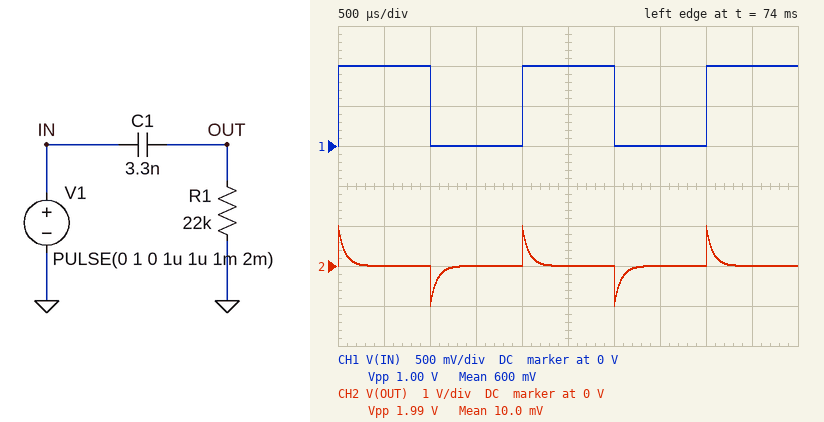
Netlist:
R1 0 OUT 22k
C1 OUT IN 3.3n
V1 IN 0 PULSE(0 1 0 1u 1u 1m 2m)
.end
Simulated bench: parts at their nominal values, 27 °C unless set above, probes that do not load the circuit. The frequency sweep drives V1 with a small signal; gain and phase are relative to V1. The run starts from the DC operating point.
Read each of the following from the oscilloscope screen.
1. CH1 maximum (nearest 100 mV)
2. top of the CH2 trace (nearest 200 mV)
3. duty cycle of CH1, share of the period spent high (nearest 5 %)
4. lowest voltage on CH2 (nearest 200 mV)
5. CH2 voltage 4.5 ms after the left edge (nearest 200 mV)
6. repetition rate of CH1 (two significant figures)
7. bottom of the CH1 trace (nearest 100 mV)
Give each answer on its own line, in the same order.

1.0 V
1.0 V
50 %
-1.0 V
0 V
500 Hz
0 V
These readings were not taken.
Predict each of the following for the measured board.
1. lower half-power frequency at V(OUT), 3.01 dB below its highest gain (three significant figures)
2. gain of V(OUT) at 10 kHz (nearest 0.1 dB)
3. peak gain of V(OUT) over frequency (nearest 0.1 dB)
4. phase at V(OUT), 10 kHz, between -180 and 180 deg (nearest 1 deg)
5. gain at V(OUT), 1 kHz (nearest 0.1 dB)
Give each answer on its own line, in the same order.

2.19 kHz
-0.2 dB
0 dB
12 deg
-7.6 dB
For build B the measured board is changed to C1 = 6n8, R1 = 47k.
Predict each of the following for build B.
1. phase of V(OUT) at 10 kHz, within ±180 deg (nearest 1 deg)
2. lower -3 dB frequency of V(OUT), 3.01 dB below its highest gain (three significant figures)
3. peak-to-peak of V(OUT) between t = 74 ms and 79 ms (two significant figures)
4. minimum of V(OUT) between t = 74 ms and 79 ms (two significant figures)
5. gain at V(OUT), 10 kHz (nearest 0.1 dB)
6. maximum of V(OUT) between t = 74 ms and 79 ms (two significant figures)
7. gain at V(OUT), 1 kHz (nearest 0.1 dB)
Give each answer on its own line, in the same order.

3 deg
498 Hz
1.9 V
-960 mV
0 dB
960 mV
-1.0 dB
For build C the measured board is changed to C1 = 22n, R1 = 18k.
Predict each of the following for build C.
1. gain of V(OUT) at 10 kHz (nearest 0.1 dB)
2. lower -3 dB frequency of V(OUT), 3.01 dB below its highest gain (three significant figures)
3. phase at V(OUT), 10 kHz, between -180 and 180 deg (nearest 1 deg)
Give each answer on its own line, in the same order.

0 dB
402 Hz
2 deg
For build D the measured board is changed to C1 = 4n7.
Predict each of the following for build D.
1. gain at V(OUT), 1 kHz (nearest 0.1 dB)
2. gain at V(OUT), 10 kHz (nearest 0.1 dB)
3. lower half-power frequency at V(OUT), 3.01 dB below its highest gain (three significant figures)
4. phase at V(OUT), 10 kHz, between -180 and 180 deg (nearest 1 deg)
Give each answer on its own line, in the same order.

-5.3 dB
-0.1 dB
1.54 kHz
9 deg
